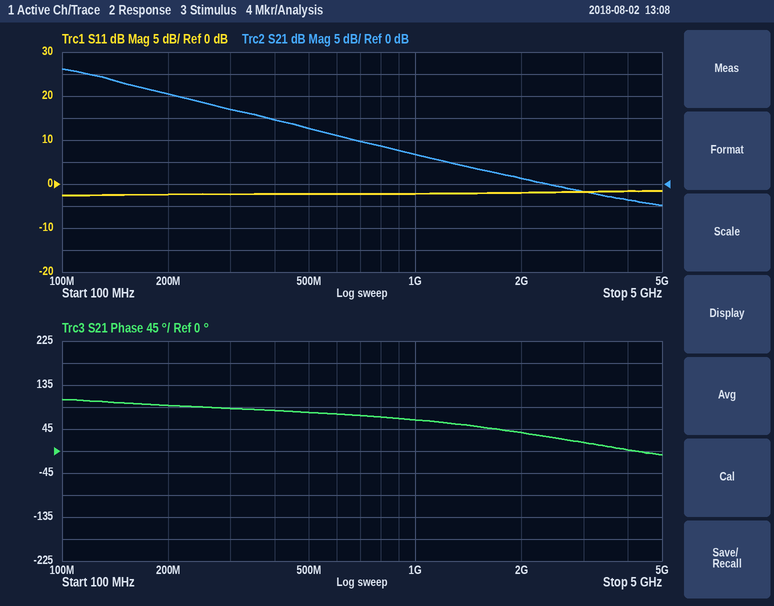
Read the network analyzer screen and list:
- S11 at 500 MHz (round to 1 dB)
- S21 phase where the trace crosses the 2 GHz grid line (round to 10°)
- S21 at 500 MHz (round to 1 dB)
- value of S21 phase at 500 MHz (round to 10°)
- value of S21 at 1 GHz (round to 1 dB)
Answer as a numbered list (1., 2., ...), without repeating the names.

1. -2 dB
2. 40°
3. 13 dB
4. 80°
5. 7 dB
